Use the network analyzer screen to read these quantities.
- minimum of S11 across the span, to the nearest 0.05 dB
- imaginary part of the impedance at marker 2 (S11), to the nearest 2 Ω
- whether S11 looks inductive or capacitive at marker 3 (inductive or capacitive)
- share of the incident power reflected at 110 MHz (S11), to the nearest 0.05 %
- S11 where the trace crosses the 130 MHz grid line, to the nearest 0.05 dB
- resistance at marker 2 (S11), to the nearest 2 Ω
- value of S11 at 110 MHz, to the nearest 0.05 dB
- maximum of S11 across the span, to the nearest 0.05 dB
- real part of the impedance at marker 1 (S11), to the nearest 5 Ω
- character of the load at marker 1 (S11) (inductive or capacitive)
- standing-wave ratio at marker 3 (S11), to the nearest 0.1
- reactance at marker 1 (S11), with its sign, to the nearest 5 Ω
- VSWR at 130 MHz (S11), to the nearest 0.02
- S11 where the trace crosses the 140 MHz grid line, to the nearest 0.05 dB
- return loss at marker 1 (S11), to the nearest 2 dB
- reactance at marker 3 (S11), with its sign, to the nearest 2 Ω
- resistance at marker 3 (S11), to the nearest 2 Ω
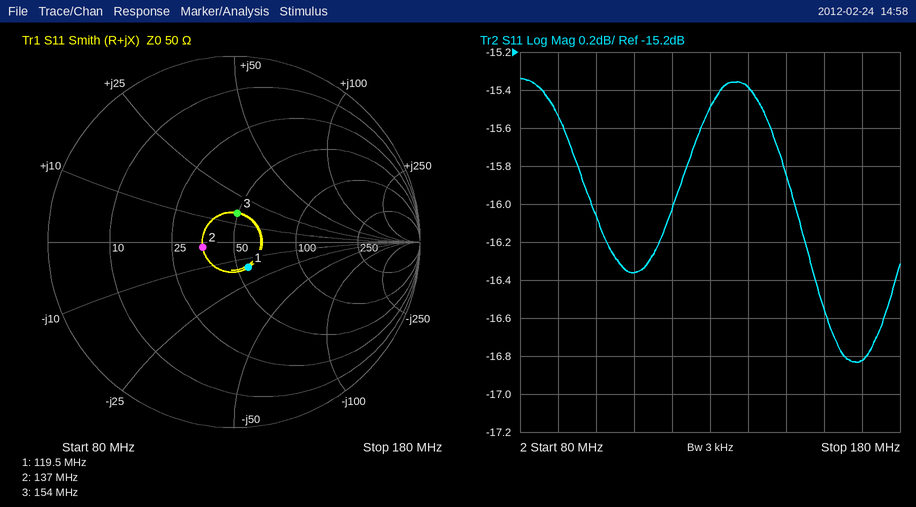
-16.85 dB
-2 Ω
inductive
2.30 %
-15.50 dB
36 Ω
-16.35 dB
-15.35 dB
55 Ω
capacitive
1.4
-15 Ω
1.40
-15.40 dB
16 dB
+16 Ω
50 Ω
